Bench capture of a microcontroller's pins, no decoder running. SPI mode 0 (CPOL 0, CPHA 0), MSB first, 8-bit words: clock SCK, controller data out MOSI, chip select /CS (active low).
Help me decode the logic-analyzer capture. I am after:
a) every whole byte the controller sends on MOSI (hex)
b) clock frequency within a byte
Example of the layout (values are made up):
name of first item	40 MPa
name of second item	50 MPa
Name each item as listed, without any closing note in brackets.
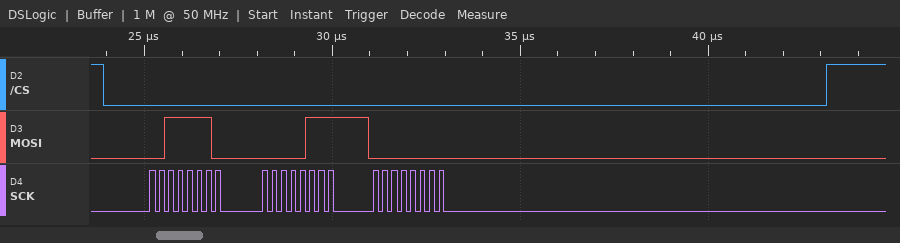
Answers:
every whole byte the controller sends on MOSI	3E 07 00
clock frequency within a byte	4 MHz
